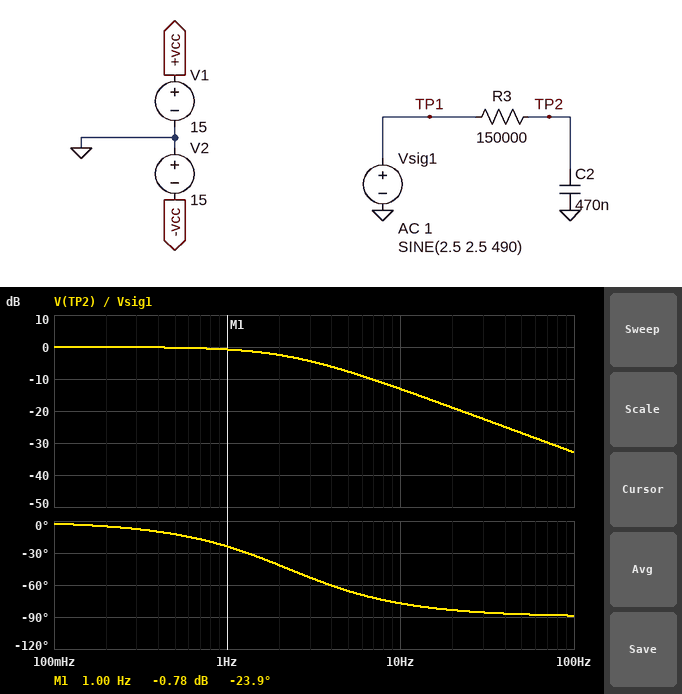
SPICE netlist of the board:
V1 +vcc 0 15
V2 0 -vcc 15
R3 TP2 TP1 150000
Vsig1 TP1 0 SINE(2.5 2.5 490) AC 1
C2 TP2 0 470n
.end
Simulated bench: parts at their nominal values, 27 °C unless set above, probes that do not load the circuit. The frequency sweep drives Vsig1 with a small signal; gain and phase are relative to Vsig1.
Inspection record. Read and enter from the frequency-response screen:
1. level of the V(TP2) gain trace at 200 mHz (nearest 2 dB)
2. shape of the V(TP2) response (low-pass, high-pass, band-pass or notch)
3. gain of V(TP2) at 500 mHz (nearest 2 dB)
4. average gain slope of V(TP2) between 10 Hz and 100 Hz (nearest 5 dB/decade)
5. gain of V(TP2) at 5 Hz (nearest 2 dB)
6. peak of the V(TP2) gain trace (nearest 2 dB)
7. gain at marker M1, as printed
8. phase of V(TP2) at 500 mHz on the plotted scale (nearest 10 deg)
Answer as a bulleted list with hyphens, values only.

- 0 dB
- low-pass
- 0 dB
- -20 dB/decade
- -8 dB
- 0 dB
- -0.78 dB
- -10 deg
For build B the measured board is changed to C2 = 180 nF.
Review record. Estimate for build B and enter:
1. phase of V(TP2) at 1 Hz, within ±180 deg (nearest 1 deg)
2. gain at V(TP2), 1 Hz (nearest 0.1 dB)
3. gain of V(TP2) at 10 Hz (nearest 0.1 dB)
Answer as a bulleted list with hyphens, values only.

- -10 deg
- -0.1 dB
- -5.9 dB
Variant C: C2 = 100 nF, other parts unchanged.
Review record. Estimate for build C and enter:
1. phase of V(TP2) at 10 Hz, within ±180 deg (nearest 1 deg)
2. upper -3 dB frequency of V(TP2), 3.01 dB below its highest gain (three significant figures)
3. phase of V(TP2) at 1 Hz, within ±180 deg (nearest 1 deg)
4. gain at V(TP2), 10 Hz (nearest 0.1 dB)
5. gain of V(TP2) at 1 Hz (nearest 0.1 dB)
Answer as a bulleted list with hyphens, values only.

- -43 deg
- 10.6 Hz
- -5 deg
- -2.8 dB
- 0 dB
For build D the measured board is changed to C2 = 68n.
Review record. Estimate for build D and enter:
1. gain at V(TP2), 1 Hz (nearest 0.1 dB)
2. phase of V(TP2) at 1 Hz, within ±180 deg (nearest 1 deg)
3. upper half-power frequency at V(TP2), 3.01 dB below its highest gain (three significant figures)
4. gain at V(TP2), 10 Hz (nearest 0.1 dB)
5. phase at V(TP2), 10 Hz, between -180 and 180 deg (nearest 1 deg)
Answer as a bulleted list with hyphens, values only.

- 0 dB
- -4 deg
- 15.6 Hz
- -1.5 dB
- -33 deg
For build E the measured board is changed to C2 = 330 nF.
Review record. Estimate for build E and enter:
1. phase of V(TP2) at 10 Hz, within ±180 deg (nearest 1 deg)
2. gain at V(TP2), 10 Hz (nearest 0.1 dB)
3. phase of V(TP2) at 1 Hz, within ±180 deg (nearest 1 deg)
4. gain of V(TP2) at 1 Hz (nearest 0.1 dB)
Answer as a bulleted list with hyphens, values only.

- -72 deg
- -10.3 dB
- -17 deg
- -0.4 dB
